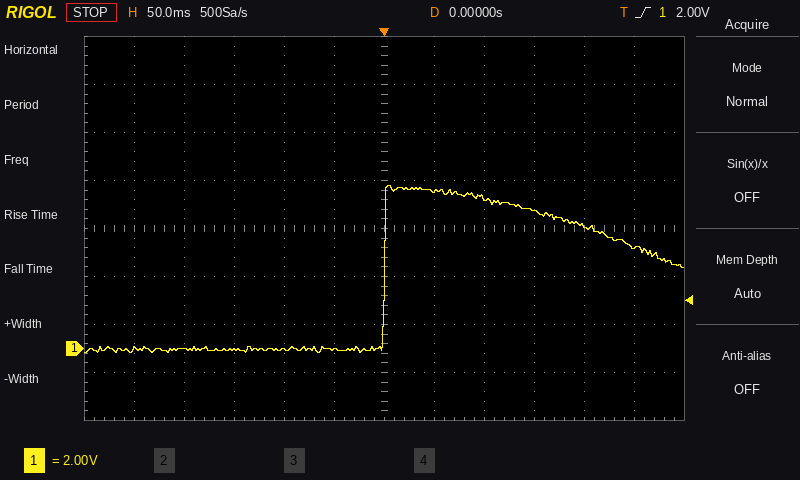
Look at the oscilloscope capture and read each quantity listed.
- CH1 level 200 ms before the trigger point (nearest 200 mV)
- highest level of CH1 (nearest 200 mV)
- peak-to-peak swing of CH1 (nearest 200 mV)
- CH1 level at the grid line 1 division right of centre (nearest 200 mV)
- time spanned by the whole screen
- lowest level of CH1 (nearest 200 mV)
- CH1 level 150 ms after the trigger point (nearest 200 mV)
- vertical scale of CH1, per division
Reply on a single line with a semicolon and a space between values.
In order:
0.0 V; 6.8 V; 7.0 V; 6.6 V; 600 ms; -200 mV; 5.8 V; 2 V
